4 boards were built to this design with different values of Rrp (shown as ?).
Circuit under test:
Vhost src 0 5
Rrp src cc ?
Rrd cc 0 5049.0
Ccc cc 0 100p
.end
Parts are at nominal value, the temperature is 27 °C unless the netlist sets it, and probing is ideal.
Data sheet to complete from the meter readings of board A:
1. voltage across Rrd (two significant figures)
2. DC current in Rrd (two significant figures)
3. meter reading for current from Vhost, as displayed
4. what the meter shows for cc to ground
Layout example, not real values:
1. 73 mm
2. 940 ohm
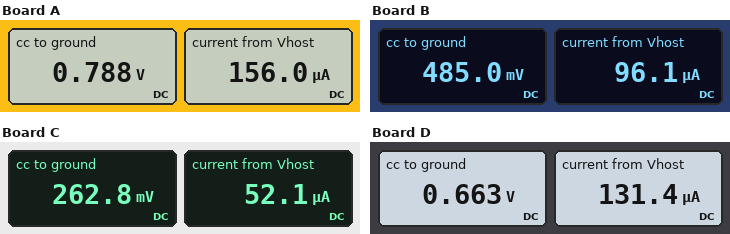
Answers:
1. 790 mV
2. 160 µA
3. 156.0 µA
4. 0.788 V
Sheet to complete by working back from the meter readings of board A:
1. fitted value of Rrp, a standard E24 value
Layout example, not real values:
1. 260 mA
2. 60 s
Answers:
1. 27 kΩ
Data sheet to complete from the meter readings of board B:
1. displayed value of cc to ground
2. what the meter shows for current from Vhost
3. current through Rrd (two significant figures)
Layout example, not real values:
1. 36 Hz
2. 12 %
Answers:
1. 485.0 mV
2. 96.1 µA
3. 96 µA
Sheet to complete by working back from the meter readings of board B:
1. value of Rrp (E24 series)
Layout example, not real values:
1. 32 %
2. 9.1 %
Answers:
1. 47 kΩ
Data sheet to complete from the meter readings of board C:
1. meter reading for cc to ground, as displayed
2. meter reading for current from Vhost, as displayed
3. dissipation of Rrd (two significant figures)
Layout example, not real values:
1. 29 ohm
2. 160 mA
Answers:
1. 262.8 mV
2. 52.1 µA
3. 14 µW
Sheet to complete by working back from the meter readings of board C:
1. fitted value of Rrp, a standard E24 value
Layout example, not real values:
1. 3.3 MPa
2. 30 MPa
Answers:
1. 91 kΩ
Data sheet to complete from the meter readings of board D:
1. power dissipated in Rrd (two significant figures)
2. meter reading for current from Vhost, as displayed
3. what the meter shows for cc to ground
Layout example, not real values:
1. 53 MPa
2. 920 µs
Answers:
1. 87 µW
2. 131.4 µA
3. 0.663 V
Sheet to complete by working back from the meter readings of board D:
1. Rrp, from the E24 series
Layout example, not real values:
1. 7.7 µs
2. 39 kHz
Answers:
1. 33 kΩ
